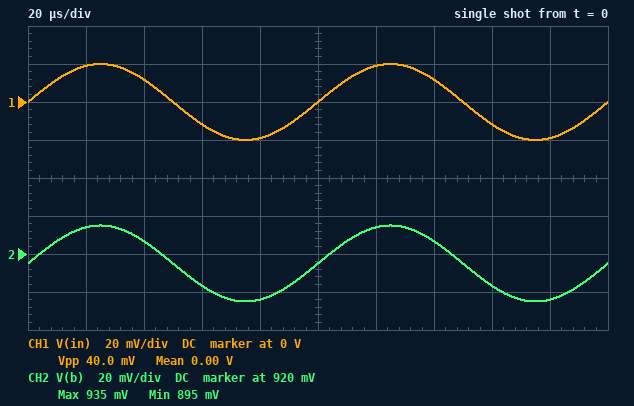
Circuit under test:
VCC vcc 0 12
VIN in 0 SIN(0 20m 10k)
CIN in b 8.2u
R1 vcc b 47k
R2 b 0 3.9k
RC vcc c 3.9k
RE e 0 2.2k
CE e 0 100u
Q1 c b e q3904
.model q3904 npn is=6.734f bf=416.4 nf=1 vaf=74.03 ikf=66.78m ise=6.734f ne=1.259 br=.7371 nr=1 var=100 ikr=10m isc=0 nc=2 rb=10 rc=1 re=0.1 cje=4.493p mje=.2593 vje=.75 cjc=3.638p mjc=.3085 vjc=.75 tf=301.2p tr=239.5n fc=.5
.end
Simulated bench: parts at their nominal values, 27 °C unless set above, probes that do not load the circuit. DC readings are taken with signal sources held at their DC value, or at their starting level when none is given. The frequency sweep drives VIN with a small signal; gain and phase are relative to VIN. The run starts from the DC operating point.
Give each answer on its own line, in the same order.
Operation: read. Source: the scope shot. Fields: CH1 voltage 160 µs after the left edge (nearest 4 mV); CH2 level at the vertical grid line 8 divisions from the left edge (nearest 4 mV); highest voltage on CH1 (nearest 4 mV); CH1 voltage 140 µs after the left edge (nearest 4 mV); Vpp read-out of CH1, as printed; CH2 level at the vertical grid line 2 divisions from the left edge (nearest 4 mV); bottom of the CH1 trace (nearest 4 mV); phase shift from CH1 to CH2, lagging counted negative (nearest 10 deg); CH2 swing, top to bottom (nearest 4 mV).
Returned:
-12 mV
904 mV
20 mV
12 mV
40.0 mV
928 mV
-20 mV
0 deg
40 mV
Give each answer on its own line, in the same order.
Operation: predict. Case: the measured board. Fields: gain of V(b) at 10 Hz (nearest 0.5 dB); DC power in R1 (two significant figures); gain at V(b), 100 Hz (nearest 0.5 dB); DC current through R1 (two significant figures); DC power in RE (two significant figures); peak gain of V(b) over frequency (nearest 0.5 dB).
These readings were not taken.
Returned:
-1.5 dB
2.6 mW
0 dB
240 µA
42 µW
0 dB
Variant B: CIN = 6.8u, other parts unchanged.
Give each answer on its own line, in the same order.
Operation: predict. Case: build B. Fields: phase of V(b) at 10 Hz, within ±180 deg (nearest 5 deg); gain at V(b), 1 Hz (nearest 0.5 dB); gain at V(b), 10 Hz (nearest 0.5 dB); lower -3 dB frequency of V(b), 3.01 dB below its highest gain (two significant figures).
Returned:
35 deg
-16.5 dB
-2.0 dB
7.4 Hz
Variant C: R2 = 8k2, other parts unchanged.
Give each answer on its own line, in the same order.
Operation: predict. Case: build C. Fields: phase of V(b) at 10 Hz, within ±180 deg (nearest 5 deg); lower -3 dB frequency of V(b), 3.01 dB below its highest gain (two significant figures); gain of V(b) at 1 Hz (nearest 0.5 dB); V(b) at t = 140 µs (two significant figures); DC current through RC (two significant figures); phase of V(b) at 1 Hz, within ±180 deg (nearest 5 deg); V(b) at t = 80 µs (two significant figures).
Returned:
15 deg
3.1 Hz
-9.5 dB
1.8 V
500 µA
70 deg
1.7 V
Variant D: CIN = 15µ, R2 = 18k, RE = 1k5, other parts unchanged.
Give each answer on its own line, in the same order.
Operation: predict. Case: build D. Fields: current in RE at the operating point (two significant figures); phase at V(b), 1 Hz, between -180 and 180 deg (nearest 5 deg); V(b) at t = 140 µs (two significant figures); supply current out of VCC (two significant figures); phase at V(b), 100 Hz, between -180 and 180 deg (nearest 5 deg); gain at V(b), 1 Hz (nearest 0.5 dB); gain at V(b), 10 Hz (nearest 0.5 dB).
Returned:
1.7 mA
40 deg
3.2 V
1.8 mA
0 deg
-2.5 dB
-0.5 dB
